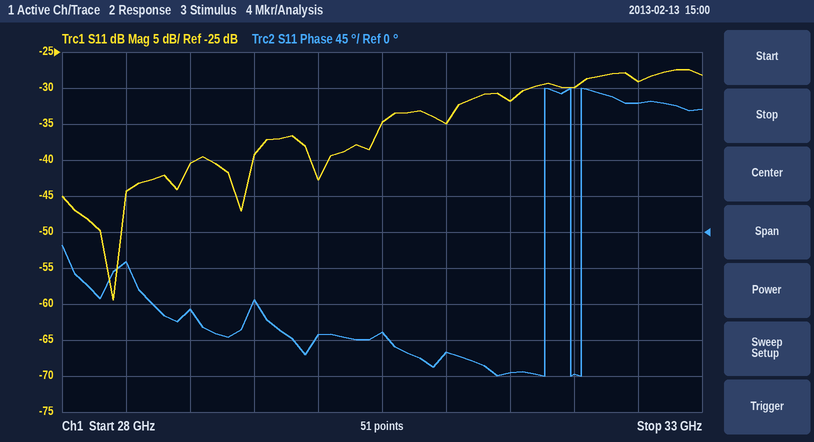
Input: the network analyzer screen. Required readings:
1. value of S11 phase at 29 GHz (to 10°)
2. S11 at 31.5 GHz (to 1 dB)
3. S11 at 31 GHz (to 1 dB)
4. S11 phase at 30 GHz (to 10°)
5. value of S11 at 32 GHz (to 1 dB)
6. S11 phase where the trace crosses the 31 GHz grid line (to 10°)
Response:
-100°
-32 dB
-35 dB
-130°
-30 dB
-150°
